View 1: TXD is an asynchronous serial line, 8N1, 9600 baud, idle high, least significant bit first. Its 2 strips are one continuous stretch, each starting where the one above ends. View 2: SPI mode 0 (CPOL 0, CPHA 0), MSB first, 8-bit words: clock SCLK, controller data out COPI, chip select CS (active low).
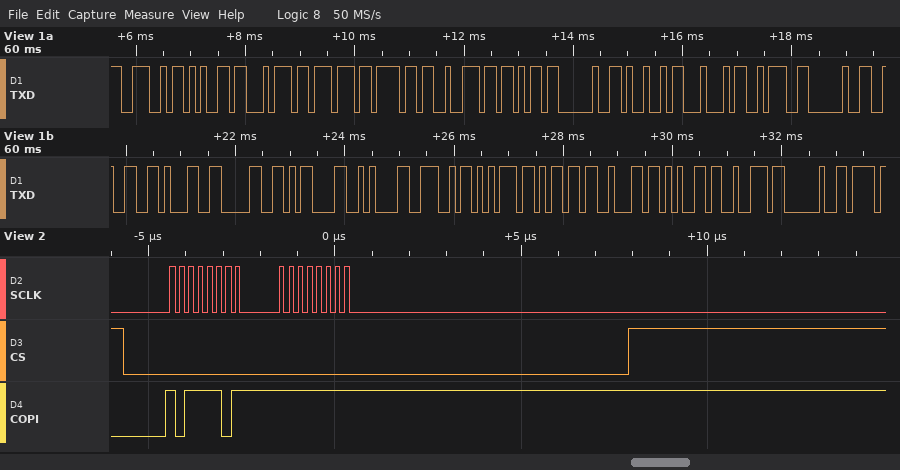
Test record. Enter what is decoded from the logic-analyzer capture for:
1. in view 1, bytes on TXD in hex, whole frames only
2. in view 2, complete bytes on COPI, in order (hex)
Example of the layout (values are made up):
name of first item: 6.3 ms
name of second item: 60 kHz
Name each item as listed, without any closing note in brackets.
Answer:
in view 1, bytes on TXD in hex, whole frames only: 0x4E 0x65 0x74 0x77 0x6F 0x72 0x6B 0x20 0x49 0x44 0x3A 0x20 0x32 0x31 0x30 0x0D 0x0A 0x4E 0x75 0x6D 0x62 0x65 0x72 0x20
in view 2, complete bytes on COPI, in order: BD FF
